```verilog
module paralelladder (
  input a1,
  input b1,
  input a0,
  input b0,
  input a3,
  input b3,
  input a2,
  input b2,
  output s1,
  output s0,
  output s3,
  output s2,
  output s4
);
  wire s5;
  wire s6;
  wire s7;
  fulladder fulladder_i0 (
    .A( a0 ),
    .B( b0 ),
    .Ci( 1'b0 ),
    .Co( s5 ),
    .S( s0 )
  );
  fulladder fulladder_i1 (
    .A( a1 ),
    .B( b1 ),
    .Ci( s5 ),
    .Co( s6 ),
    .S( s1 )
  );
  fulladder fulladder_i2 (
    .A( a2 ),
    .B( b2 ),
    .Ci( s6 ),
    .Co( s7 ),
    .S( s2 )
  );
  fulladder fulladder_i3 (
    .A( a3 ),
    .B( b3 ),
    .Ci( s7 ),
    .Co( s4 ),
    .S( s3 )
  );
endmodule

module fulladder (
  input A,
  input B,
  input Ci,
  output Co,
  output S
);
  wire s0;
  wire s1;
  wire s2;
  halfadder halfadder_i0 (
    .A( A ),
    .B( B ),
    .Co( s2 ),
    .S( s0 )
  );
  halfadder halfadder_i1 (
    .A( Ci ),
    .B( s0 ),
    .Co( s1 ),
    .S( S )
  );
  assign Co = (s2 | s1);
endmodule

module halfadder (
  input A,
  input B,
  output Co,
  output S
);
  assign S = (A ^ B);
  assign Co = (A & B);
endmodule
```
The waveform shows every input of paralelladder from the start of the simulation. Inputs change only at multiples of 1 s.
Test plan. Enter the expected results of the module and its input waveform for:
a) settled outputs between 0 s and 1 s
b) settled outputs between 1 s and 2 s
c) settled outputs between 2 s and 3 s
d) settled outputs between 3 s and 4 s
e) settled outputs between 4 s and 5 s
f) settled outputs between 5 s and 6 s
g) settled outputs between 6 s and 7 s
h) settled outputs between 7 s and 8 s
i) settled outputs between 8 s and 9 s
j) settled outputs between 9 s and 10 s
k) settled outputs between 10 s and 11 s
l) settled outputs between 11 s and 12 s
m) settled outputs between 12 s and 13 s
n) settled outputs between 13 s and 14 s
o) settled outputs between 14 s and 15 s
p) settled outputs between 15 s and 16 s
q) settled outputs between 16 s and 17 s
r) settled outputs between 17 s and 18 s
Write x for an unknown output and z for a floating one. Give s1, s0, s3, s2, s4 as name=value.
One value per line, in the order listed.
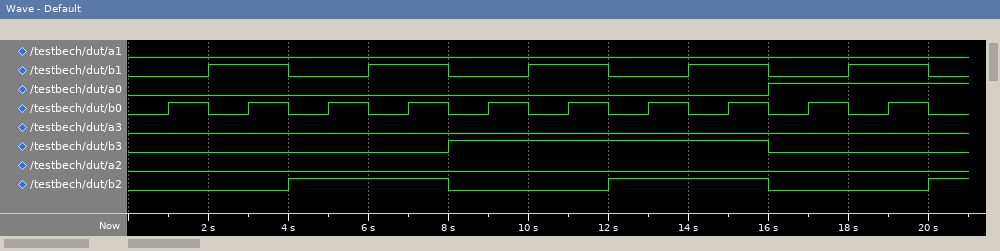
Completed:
s1=0, s0=0, s3=0, s2=0, s4=0
s1=0, s0=1, s3=0, s2=0, s4=0
s1=1, s0=0, s3=0, s2=0, s4=0
s1=1, s0=1, s3=0, s2=0, s4=0
s1=0, s0=0, s3=0, s2=1, s4=0
s1=0, s0=1, s3=0, s2=1, s4=0
s1=1, s0=0, s3=0, s2=1, s4=0
s1=1, s0=1, s3=0, s2=1, s4=0
s1=0, s0=0, s3=1, s2=0, s4=0
s1=0, s0=1, s3=1, s2=0, s4=0
s1=1, s0=0, s3=1, s2=0, s4=0
s1=1, s0=1, s3=1, s2=0, s4=0
s1=0, s0=0, s3=1, s2=1, s4=0
s1=0, s0=1, s3=1, s2=1, s4=0
s1=1, s0=0, s3=1, s2=1, s4=0
s1=1, s0=1, s3=1, s2=1, s4=0
s1=0, s0=1, s3=0, s2=0, s4=0
s1=1, s0=0, s3=0, s2=0, s4=0
